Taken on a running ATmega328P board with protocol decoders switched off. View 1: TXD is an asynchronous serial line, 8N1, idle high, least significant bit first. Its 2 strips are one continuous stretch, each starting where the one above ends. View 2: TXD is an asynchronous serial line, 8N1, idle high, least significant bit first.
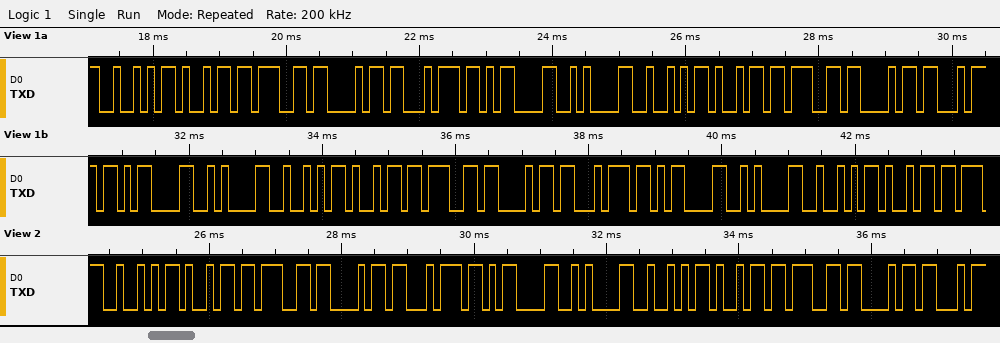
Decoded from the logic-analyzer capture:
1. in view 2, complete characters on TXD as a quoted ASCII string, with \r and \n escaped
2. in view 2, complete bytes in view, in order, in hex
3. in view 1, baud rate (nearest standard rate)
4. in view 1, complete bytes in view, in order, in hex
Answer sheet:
"Right\r\nRigh"
52 69 67 68 74 0D 0A 52 69 67 68
9600 baud
0x52 0x69 0x67 0x68 0x74 0x0D 0x0A 0x52 0x69 0x67 0x68 0x74 0x0D 0x0A 0x52 0x69 0x67 0x68 0x74 0x0D 0x0A 0x52 0x69
